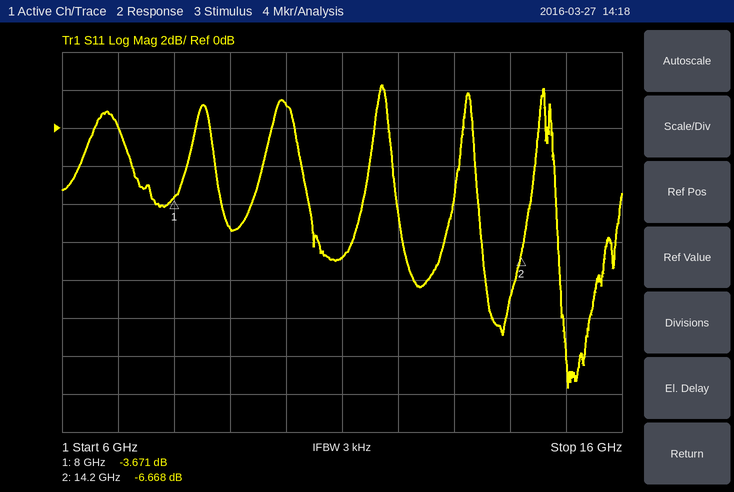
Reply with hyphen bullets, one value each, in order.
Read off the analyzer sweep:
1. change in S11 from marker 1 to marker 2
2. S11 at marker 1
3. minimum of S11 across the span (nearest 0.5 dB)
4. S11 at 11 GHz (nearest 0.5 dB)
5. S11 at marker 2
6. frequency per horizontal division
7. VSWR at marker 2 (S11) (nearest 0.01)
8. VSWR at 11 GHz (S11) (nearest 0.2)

- -2.997 dB
- -3.671 dB
- -13.5 dB
- -7.0 dB
- -6.668 dB
- 1 GHz
- 2.73
- 2.6
